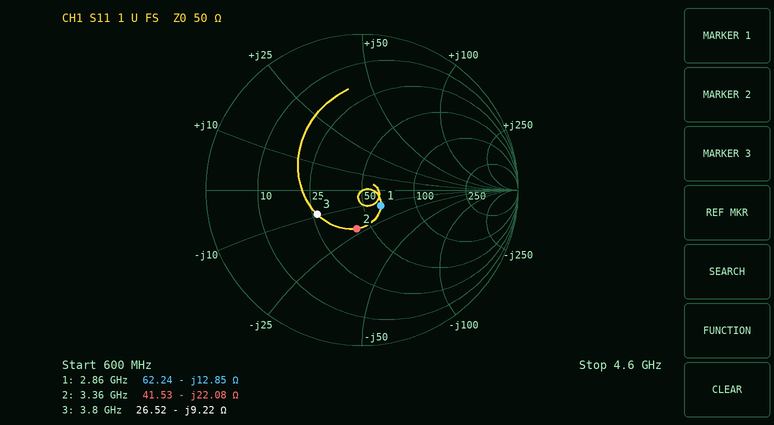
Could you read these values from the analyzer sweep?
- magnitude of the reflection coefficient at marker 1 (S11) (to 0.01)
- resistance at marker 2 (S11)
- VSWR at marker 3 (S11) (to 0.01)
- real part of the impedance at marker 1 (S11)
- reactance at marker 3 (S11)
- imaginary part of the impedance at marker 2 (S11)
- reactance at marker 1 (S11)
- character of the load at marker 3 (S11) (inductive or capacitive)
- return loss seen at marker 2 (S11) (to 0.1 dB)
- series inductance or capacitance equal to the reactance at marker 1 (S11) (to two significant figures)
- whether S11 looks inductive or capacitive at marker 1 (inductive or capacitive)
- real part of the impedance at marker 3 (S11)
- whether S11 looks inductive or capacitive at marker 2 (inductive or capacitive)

0.16
41.53 Ω
1.97
62.24 Ω
-9.22 Ω
-22.08 Ω
-12.85 Ω
capacitive
12.0 dB
4.3 pF
capacitive
26.52 Ω
capacitive
